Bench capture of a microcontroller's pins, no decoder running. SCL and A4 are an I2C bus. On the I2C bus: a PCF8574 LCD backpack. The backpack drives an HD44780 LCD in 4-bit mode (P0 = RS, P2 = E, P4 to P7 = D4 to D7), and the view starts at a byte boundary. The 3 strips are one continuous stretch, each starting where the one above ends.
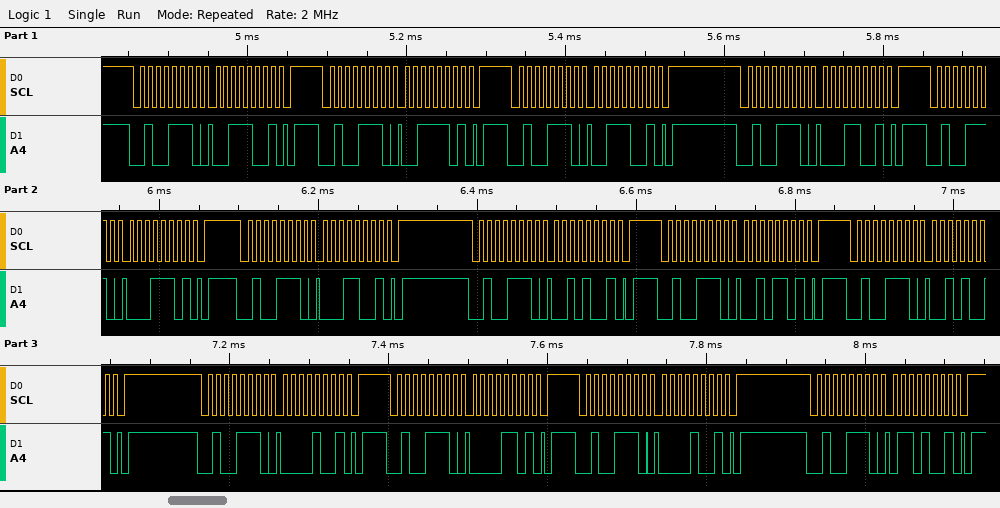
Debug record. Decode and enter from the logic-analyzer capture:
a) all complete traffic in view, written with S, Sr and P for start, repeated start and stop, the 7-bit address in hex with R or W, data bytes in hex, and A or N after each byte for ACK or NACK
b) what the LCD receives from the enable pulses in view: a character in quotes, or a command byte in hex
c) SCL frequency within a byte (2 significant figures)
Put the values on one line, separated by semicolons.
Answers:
S 27W A 39 A P S 27W A 3D A P S 27W A 39 A P S 27W A 19 A P S 27W A 1D A P S 27W A 19 A P S 27W A 29 A P S 27W A 2D A P S 27W A 29 A P S 27W A 09 A P S 27W A 0D A P S 27W A 09 A P S 27W A 69 A P; '1' ' '; 100 kHz
